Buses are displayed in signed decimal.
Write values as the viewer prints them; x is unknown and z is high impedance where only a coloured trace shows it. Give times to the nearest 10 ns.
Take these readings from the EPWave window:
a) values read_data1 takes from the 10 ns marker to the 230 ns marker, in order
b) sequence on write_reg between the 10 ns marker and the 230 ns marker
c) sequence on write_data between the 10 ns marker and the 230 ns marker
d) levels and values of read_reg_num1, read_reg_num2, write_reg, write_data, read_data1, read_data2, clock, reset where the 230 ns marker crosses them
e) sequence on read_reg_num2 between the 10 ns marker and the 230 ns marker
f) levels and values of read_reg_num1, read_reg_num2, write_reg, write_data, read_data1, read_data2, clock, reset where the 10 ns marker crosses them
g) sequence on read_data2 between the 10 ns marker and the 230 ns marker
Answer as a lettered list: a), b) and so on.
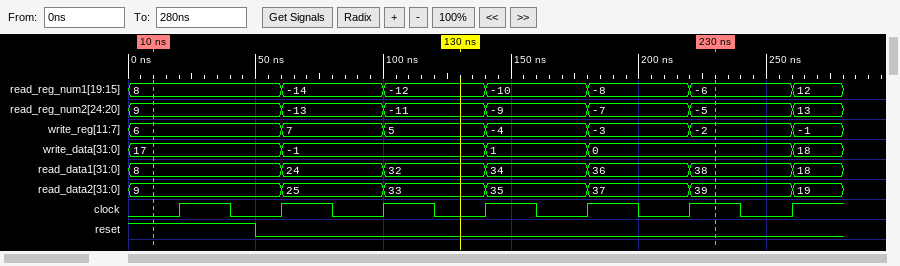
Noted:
a) 8, 24, 32, 34, 36, 38
b) 6, 7, 5, -4, -3, -2
c) 17, -1, 1, 0
d) read_reg_num1=-6, read_reg_num2=-5, write_reg=-2, write_data=0, read_data1=38, read_data2=39, clock=1, reset=0
e) 9, -13, -11, -9, -7, -5
f) read_reg_num1=8, read_reg_num2=9, write_reg=6, write_data=17, read_data1=8, read_data2=9, clock=0, reset=1
g) 9, 25, 33, 35, 37, 39
